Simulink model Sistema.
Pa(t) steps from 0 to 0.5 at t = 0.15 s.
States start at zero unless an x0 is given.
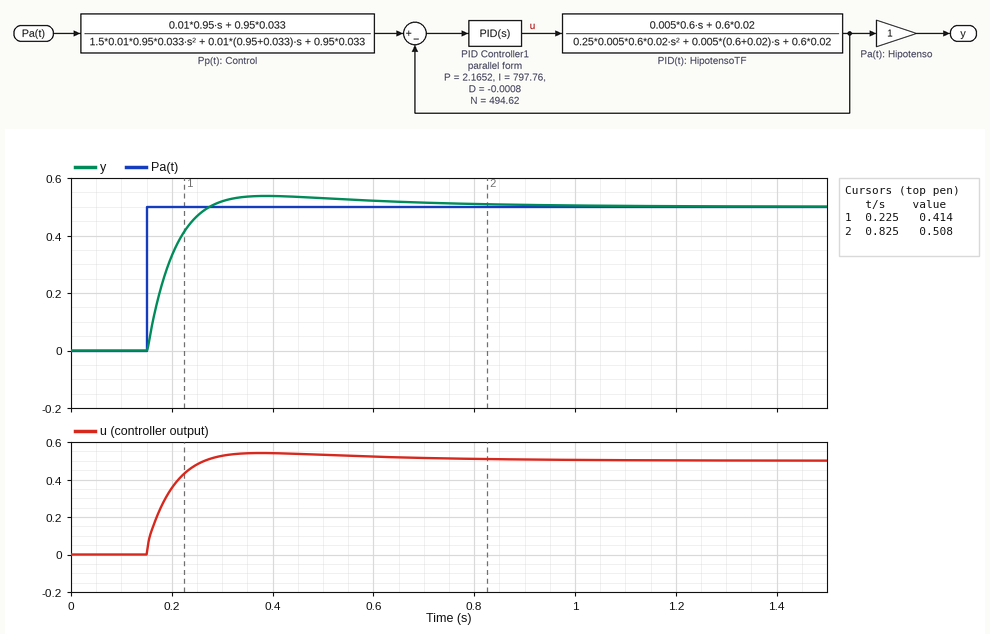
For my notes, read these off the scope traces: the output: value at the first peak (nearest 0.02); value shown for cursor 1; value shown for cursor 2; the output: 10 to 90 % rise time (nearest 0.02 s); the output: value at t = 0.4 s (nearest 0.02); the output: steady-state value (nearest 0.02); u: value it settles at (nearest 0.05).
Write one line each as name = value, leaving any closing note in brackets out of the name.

the output: value at the first peak = 0.54
value shown for cursor 1 = 0.414
value shown for cursor 2 = 0.508
the output: 10 to 90 % rise time = 0.08 s
the output: value at t = 0.4 s = 0.54
the output: steady-state value = 0.50
u: value it settles at = 0.50
